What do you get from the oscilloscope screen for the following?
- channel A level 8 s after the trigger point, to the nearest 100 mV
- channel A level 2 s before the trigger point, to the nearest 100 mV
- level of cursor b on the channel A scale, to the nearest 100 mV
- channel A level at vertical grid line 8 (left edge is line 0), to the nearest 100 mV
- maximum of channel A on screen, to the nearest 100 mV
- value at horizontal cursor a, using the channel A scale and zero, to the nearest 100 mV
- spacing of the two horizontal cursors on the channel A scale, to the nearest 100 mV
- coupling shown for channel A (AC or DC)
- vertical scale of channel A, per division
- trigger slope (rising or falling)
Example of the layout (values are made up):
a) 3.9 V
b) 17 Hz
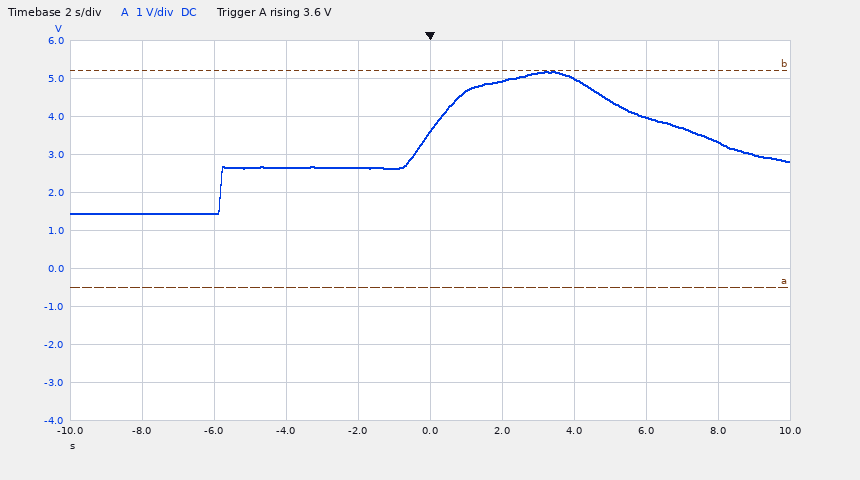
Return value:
a) 3.3 V
b) 2.7 V
c) 5.2 V
d) 4.0 V
e) 5.2 V
f) -500 mV
g) 5.7 V
h) DC
i) 1 V
j) rising
